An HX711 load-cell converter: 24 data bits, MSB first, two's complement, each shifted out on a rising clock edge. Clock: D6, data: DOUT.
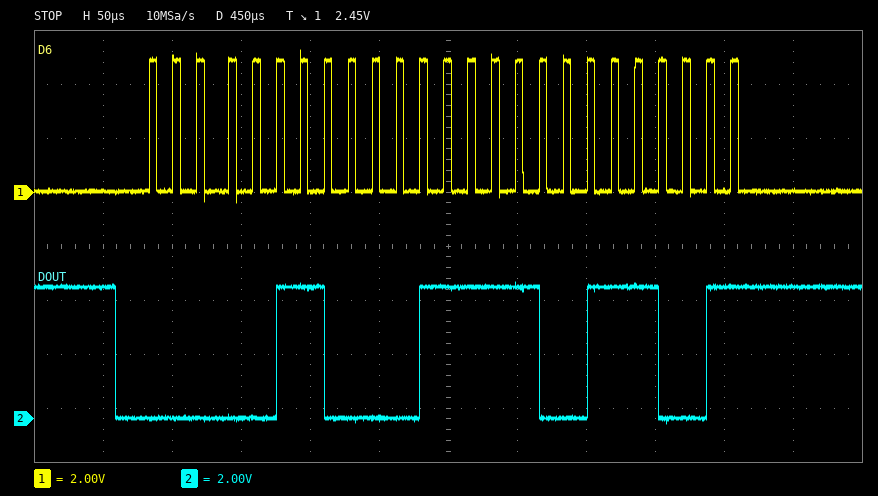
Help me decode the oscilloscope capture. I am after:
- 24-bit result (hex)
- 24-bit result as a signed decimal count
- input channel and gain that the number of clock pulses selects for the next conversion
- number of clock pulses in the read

0x061F39
401209
channel A, gain 128
25
